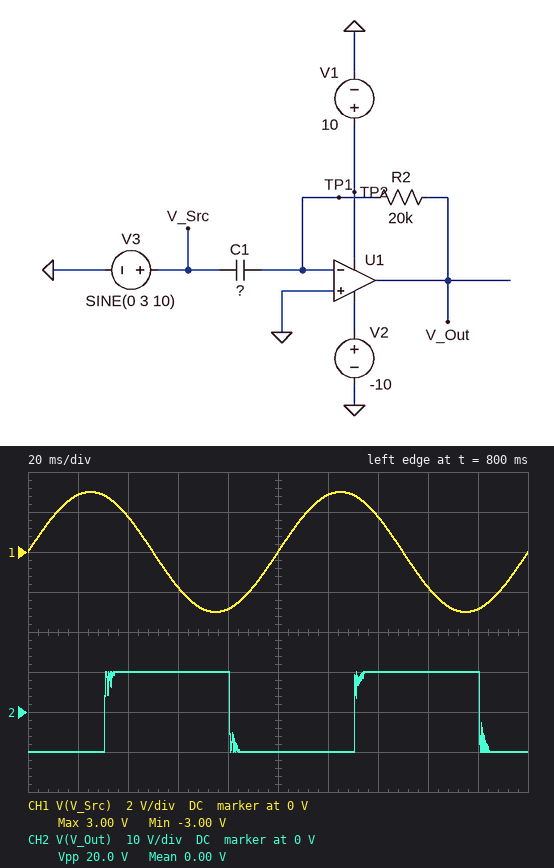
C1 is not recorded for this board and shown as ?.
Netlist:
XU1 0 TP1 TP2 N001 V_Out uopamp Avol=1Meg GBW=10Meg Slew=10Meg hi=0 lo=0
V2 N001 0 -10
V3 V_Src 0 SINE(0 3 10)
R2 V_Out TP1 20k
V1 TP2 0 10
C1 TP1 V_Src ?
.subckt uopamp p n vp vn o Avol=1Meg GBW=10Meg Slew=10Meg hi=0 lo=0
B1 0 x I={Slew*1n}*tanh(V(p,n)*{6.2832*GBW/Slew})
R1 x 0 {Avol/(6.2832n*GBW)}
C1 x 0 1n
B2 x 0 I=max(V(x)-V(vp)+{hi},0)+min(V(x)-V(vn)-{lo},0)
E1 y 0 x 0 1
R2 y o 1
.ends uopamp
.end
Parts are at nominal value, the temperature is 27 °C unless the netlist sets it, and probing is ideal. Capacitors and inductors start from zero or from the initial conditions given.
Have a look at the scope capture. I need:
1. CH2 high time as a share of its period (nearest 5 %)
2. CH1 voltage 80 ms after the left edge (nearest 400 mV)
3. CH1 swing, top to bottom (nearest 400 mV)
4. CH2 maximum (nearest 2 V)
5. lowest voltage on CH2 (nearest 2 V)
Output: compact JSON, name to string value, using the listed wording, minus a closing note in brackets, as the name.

{"CH2 high time as a share of its period": "50 %", "CH1 voltage 80 ms after the left edge": "-2.8 V", "CH1 swing, top to bottom": "6.0 V", "CH2 maximum": "10 V", "lowest voltage on CH2": "-10 V"}
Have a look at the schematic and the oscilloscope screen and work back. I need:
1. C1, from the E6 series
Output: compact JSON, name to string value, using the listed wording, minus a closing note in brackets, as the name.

{"C1, from the E6 series": "4.7 µF"}
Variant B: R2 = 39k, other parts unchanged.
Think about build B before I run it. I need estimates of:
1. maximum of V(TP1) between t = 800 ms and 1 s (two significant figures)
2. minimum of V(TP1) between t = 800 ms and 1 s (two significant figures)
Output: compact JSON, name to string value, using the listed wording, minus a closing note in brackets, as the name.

{"maximum of V(TP1) between t = 800 ms and 1 s": "2.6 V", "minimum of V(TP1) between t = 800 ms and 1 s": "-2.6 V"}
